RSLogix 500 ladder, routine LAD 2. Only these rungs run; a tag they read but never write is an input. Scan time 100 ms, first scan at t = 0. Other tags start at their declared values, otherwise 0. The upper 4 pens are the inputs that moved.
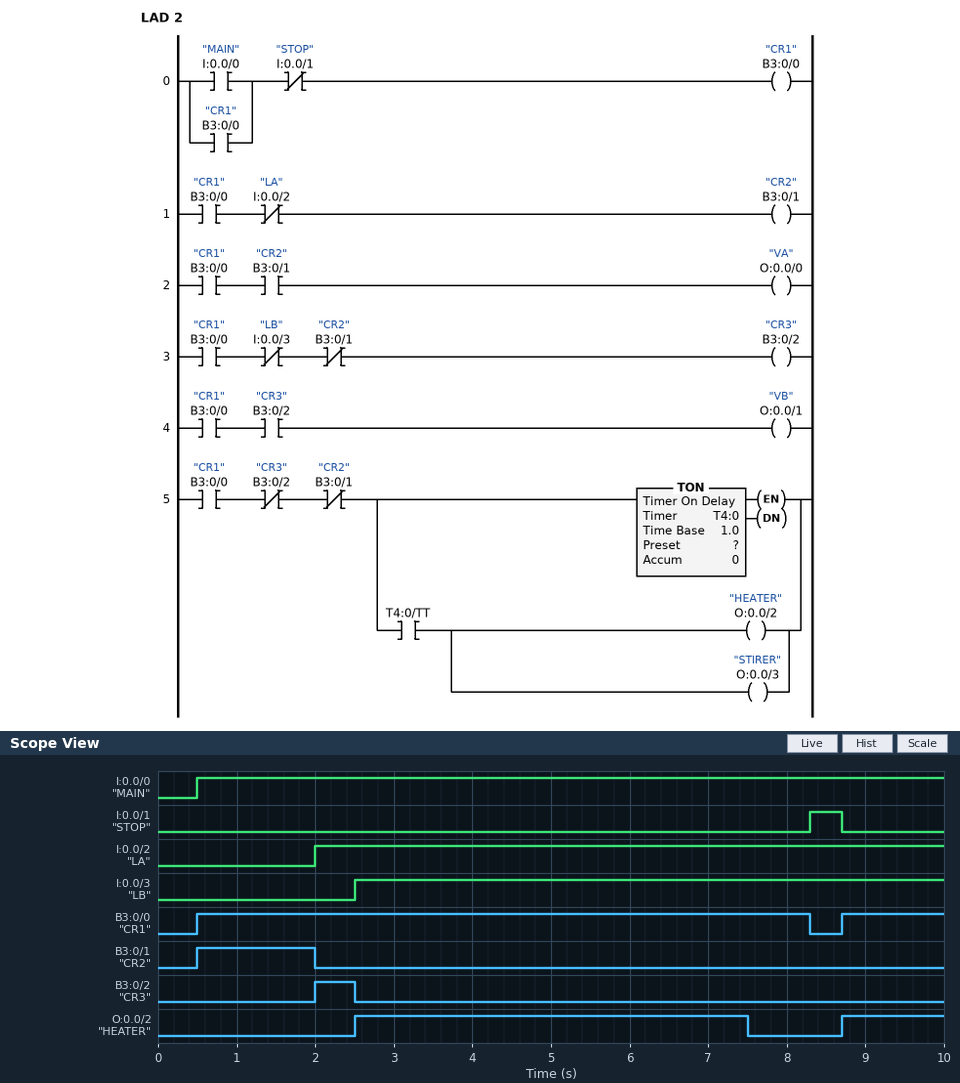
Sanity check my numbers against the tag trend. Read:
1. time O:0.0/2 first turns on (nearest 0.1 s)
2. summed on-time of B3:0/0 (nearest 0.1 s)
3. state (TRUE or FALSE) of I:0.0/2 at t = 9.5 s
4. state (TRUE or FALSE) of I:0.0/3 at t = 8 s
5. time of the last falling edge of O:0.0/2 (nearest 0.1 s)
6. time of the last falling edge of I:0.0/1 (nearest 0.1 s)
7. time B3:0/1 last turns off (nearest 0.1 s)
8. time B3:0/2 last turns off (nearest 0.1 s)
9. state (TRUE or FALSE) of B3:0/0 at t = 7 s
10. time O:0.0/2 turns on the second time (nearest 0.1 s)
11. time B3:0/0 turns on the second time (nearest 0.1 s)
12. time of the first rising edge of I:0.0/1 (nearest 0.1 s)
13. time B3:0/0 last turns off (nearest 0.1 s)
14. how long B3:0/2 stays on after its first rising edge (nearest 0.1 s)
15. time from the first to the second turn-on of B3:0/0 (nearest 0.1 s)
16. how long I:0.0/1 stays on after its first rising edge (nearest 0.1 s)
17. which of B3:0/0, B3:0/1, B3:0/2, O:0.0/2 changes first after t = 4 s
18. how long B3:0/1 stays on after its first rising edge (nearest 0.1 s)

2.5 s
9.1 s
TRUE
TRUE
7.5 s
8.7 s
2.0 s
2.5 s
TRUE
8.7 s
8.7 s
8.3 s
8.3 s
0.5 s
8.2 s
0.4 s
O:0.0/2
1.5 s
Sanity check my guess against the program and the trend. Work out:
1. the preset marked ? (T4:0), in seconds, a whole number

5 s
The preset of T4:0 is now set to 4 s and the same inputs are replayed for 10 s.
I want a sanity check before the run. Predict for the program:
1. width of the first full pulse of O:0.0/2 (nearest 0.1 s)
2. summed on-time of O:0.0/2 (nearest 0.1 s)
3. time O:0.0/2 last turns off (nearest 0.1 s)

4.0 s
5.3 s
6.5 s
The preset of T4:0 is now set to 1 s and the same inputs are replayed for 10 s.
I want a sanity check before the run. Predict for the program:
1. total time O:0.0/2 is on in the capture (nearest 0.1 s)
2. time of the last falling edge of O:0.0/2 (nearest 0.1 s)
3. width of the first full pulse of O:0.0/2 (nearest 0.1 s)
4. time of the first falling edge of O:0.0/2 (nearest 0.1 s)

2.0 s
9.7 s
1.0 s
3.5 s
